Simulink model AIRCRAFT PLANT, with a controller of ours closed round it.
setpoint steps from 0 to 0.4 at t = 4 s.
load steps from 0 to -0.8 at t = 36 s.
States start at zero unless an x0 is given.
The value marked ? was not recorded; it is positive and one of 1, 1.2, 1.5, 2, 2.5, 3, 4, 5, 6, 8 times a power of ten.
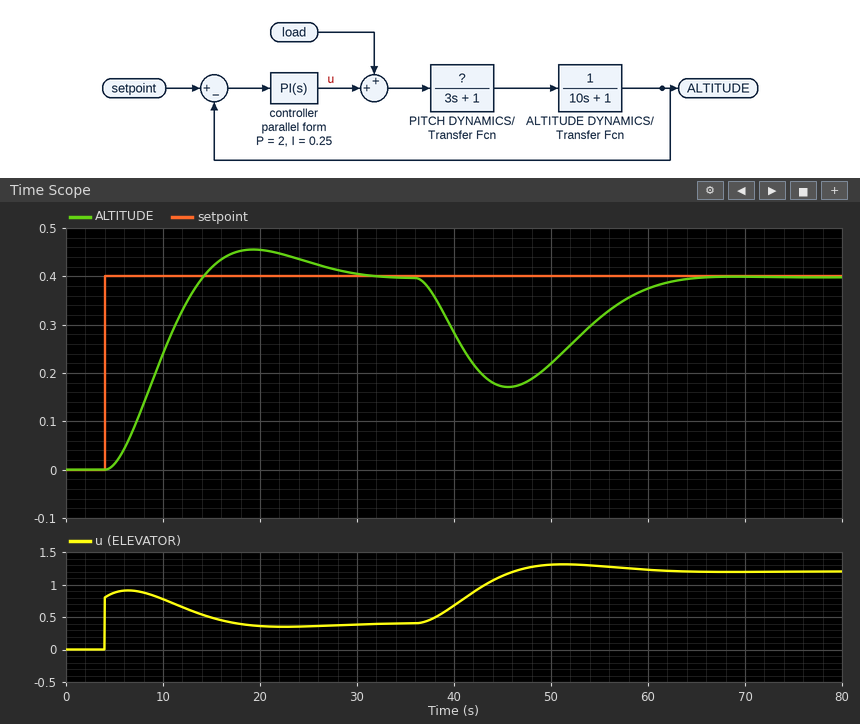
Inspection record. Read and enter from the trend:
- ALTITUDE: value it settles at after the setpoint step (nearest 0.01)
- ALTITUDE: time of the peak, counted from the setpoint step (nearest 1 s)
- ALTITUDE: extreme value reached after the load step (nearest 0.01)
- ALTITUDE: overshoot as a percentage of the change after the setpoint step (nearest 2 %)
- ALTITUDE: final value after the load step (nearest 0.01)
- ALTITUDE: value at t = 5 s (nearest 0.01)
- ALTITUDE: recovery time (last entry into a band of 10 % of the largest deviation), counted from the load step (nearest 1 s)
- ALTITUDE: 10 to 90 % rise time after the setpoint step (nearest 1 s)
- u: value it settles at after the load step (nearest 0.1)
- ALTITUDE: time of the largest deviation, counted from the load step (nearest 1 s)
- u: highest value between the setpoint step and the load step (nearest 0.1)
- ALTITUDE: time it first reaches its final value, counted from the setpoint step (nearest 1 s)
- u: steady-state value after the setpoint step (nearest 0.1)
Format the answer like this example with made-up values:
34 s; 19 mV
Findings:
0.40; 15 s; 0.17; 14 %; 0.40; 0.01; 24 s; 7 s; 1.2; 10 s; 0.9; 10 s; 0.4
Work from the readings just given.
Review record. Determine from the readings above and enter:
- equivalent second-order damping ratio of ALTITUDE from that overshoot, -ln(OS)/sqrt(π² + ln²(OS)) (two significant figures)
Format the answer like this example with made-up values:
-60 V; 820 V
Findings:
0.53
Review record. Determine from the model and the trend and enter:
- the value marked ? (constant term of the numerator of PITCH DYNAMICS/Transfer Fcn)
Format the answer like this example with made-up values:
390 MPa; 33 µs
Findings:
1
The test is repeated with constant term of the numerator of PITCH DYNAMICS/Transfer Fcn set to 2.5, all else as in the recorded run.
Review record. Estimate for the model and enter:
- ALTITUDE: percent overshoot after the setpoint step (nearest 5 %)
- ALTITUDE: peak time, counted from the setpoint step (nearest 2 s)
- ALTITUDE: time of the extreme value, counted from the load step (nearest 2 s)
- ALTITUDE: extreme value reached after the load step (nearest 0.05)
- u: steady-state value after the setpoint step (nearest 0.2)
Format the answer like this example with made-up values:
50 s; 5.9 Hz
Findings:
30 %; 8 s; 6 s; 0.05; 0.2
